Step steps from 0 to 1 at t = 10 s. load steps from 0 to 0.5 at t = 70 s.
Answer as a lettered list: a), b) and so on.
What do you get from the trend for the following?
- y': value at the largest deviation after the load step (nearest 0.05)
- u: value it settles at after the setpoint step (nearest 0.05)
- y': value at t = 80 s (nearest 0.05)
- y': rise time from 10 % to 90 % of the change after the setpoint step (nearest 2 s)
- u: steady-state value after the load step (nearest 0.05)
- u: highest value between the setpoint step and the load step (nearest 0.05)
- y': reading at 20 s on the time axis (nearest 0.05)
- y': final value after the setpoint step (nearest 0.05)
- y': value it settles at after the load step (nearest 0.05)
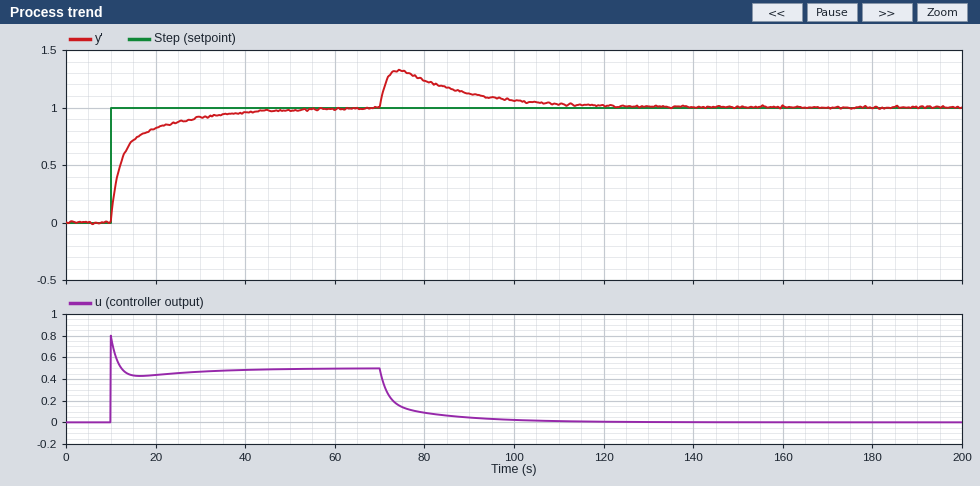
a) 1.30
b) 0.50
c) 1.25
d) 18 s
e) 0.00
f) 0.80
g) 0.80
h) 1.00
i) 1.00
